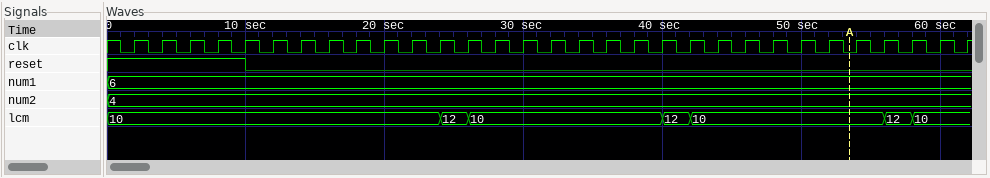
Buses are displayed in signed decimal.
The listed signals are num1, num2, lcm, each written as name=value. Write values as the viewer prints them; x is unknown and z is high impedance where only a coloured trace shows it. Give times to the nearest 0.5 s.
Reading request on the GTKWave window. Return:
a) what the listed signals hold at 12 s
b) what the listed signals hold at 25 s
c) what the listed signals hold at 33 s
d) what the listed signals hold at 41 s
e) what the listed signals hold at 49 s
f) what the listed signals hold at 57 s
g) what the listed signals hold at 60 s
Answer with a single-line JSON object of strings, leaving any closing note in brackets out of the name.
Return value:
{"what the listed signals hold at 12 s": "num1=6, num2=4, lcm=10", "what the listed signals hold at 25 s": "num1=6, num2=4, lcm=12", "what the listed signals hold at 33 s": "num1=6, num2=4, lcm=10", "what the listed signals hold at 41 s": "num1=6, num2=4, lcm=12", "what the listed signals hold at 49 s": "num1=6, num2=4, lcm=10", "what the listed signals hold at 57 s": "num1=6, num2=4, lcm=12", "what the listed signals hold at 60 s": "num1=6, num2=4, lcm=10"}
